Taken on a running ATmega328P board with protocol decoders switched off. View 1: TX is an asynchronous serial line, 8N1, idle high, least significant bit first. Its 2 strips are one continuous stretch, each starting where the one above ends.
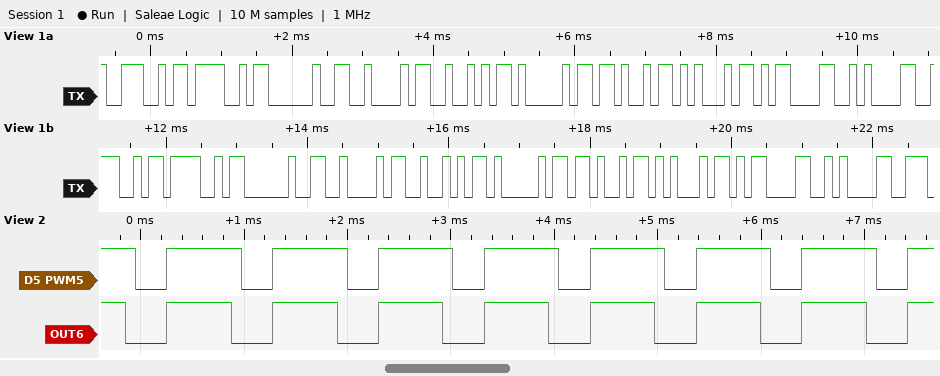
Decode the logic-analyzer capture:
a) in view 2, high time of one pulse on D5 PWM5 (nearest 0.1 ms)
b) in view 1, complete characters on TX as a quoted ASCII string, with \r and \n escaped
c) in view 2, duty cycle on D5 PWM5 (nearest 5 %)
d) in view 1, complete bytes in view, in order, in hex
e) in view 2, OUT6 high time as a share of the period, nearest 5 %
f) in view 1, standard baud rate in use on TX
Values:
0.7 ms
"NO BRAKE\r\nNO BRAKE\r\n"
70 %
4E 4F 20 42 52 41 4B 45 0D 0A 4E 4F 20 42 52 41 4B 45 0D 0A
60 %
9600 baud
